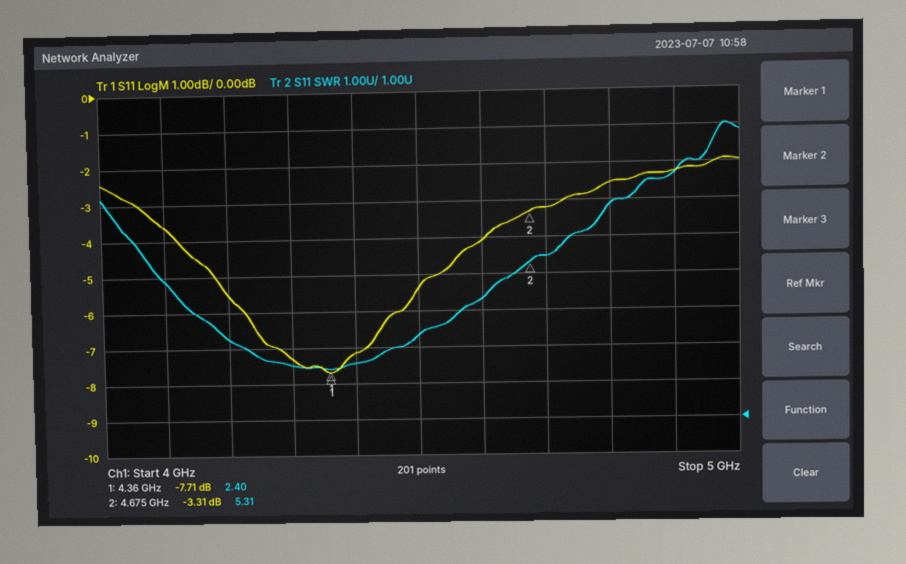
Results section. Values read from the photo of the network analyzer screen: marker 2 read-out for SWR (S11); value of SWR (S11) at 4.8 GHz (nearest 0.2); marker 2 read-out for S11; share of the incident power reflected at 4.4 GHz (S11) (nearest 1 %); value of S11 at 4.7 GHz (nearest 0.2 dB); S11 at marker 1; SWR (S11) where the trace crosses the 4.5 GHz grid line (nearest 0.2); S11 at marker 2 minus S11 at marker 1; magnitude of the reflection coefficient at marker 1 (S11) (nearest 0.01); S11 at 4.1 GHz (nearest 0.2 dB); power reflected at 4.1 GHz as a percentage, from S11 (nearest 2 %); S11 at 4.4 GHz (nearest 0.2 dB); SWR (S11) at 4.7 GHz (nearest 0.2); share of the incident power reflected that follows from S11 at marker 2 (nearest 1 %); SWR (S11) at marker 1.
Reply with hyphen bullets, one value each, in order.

- 5.31
- 6.8
- -3.31 dB
- 19 %
- -3.2 dB
- -7.71 dB
- 3.4
- 4.40 dB
- 0.41
- -3.6 dB
- 44 %
- -7.2 dB
- 5.4
- 47 %
- 2.40
